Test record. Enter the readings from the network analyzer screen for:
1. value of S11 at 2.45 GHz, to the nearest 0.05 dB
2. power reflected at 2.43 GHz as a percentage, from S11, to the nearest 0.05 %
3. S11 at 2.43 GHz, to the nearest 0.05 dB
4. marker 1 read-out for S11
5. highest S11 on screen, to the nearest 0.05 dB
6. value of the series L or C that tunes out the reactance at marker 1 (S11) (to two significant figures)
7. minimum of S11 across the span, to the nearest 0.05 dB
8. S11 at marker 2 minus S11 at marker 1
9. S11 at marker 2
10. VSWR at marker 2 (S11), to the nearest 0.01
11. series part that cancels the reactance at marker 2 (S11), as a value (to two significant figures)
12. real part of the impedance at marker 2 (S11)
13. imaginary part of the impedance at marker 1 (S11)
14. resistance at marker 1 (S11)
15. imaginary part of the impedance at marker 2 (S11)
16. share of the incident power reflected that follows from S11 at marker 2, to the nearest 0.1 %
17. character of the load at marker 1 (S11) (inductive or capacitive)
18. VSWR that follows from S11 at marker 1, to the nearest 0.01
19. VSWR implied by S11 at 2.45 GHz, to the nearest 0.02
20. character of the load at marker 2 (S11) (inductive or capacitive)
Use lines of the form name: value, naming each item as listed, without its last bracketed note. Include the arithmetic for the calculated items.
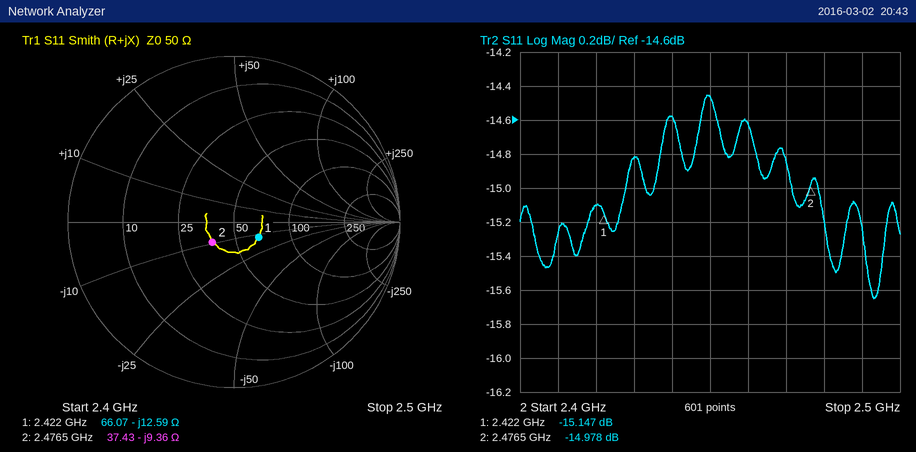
value of S11 at 2.45 GHz, to the nearest 0.05 dB: -14.45 dB
power reflected at 2.43 GHz as a percentage, from S11, to the nearest 0.05 %: 10^(-14.8/10) ≈ 3.31 %, so 3.30 % to the nearest 0.05 %
S11 at 2.43 GHz, to the nearest 0.05 dB: -14.80 dB
marker 1 read-out for S11: -15.147 dB
highest S11 on screen, to the nearest 0.05 dB: -14.45 dB
value of the series L or C that tunes out the reactance at marker 1 (S11): L = 12.59 Ω/(2π × 2.422 GHz) ≈ 827 pH, so 830 pH to two significant figures
minimum of S11 across the span, to the nearest 0.05 dB: -15.65 dB
S11 at marker 2 minus S11 at marker 1: -14.978 − (-15.147) = 0.169 dB
S11 at marker 2: -14.978 dB
VSWR at marker 2 (S11), to the nearest 0.01: 1.43
series part that cancels the reactance at marker 2 (S11), as a value: L = 9.36 Ω/(2π × 2.4765 GHz) ≈ 602 pH, so 600 pH to two significant figures
real part of the impedance at marker 2: 37.43 Ω
imaginary part of the impedance at marker 1: -12.59 Ω
resistance at marker 1: 66.07 Ω
imaginary part of the impedance at marker 2: -9.36 Ω
share of the incident power reflected that follows from S11 at marker 2, to the nearest 0.1 %: 10^(-14.978/10) ≈ 3.2 %
character of the load at marker 1 (S11): capacitive
VSWR that follows from S11 at marker 1, to the nearest 0.01: (1 + 0.1748)/(1 − 0.1748) ≈ 1.42
VSWR implied by S11 at 2.45 GHz, to the nearest 0.02: |Γ| = 10^(-14.45/20) = 0.1895; VSWR = (1 + 0.1895)/(1 − 0.1895) ≈ 1.47, so 1.46 to the nearest 0.02
character of the load at marker 2 (S11): capacitive
